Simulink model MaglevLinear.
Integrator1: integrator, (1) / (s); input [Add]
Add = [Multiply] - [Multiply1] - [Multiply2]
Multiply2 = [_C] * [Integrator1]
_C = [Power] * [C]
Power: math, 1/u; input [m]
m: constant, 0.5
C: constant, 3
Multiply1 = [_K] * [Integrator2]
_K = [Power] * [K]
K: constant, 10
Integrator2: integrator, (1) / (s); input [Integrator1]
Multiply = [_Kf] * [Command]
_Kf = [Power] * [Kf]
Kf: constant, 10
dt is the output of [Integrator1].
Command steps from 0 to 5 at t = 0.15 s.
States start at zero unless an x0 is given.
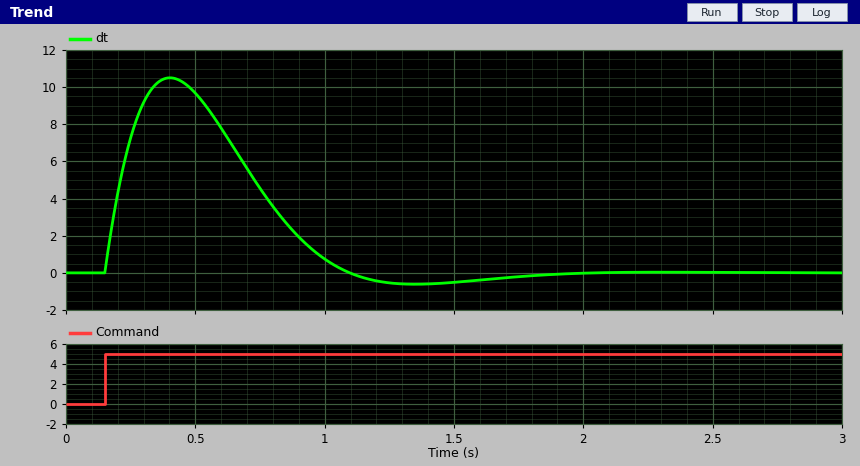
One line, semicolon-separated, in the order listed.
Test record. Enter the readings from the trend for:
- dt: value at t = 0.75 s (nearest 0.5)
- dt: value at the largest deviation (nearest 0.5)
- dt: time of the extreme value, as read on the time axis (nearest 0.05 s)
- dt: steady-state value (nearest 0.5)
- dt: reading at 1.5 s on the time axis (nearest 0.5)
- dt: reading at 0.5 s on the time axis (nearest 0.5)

4.5; 10.5; 0.40 s; 0.0; -0.5; 9.5
